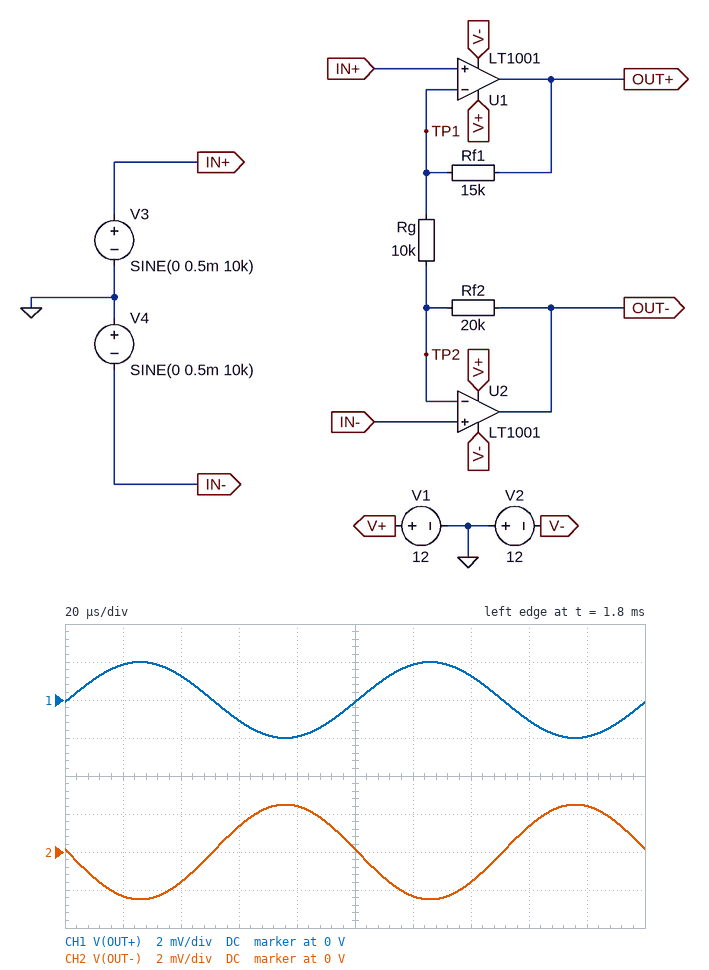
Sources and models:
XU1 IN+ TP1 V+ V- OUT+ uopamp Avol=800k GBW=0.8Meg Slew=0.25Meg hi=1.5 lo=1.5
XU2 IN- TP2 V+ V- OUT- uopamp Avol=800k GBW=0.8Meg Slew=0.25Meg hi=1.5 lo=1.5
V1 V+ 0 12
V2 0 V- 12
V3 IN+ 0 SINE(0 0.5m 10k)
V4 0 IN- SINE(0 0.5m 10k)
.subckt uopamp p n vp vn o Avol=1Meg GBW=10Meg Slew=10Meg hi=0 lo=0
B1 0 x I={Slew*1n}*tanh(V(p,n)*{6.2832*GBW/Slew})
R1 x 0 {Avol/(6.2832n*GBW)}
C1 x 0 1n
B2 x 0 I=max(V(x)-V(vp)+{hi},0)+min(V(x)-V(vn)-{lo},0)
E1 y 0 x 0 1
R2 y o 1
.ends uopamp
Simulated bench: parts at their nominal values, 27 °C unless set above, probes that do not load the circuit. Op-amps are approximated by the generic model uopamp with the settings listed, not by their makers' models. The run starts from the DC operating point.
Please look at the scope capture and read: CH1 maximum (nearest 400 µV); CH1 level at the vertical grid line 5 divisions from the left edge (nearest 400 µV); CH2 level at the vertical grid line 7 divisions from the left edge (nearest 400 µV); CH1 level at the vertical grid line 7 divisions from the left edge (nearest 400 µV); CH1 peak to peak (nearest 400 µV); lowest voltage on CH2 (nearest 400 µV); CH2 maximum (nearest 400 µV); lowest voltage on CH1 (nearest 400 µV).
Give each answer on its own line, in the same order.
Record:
2.0 mV
0 V
-1.6 mV
1.2 mV
4.0 mV
-2.4 mV
2.4 mV
-2.0 mV
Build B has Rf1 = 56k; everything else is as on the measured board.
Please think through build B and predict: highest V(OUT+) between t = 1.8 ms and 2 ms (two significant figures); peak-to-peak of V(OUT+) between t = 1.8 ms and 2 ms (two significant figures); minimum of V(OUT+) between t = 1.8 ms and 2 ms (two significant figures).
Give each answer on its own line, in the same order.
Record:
6.1 mV
12 mV
-6.1 mV
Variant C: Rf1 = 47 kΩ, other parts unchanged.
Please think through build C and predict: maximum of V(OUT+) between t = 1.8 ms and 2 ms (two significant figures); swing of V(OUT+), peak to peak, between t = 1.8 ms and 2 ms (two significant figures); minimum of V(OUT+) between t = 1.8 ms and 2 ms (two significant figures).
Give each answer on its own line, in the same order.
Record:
5.2 mV
10 mV
-5.2 mV
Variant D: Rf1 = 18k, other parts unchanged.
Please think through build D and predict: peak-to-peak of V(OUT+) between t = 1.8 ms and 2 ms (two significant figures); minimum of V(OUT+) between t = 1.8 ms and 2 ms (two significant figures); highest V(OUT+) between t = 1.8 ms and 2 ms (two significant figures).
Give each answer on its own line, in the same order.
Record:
4.6 mV
-2.3 mV
2.3 mV
